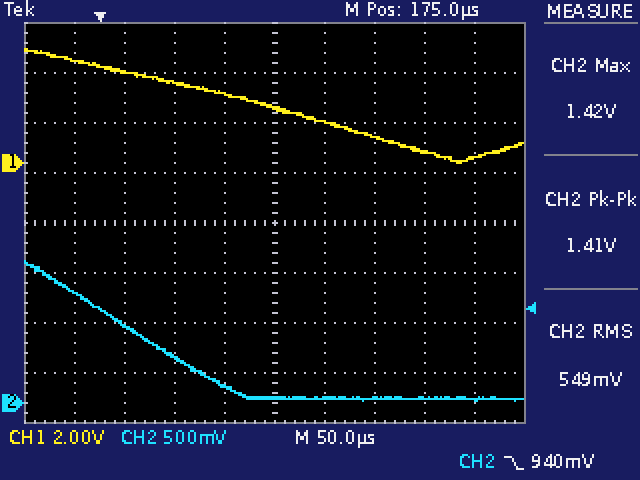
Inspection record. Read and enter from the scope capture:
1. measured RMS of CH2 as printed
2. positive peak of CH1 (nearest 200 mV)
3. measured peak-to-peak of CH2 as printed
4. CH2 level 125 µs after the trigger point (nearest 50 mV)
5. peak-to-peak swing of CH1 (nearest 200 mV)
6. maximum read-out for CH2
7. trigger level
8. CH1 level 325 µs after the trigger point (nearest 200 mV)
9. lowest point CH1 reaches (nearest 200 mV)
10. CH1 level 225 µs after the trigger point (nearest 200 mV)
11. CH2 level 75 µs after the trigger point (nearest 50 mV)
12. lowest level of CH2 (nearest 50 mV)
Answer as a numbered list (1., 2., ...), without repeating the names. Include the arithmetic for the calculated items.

1. 549 mV
2. 4.6 V
3. 1.41 V
4. 150 mV
5. 4.6 V − (0.0 V) = 4.6 V
6. 1.42 V
7. 940 mV
8. 400 mV
9. 0.0 V
10. 1.6 V
11. 450 mV
12. 0 mV
